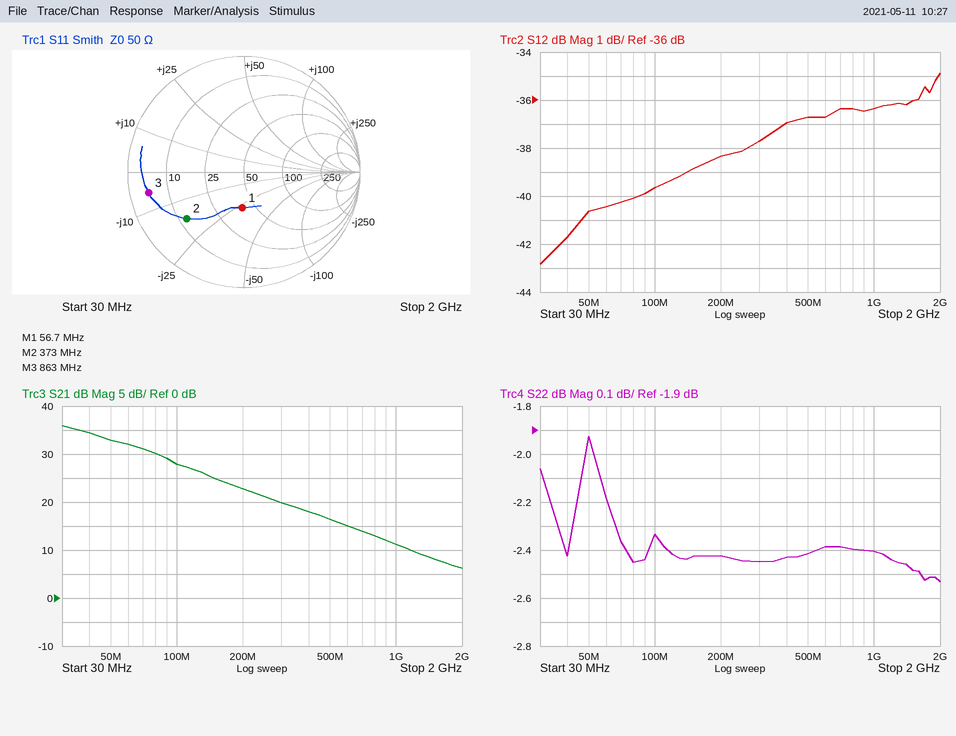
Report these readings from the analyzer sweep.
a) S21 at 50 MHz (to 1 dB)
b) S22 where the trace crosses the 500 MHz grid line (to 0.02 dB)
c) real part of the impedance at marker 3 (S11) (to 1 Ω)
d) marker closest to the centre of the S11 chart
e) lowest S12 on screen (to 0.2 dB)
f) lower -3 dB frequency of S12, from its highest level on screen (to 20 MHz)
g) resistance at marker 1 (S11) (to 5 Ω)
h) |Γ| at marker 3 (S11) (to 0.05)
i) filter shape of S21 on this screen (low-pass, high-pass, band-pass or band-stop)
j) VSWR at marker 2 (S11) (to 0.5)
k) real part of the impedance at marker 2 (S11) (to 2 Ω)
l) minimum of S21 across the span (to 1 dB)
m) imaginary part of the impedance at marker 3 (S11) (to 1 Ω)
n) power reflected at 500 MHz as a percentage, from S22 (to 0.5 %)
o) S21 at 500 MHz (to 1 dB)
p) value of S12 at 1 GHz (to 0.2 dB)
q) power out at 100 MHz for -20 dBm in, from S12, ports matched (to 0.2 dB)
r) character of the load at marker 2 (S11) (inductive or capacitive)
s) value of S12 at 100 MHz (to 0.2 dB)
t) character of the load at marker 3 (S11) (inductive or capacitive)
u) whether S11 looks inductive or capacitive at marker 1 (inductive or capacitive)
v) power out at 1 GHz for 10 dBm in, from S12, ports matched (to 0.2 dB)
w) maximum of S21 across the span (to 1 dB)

33 dB
-2.42 dB
4 Ω
marker 1
-42.8 dB
280 MHz
40 Ω
0.85
low-pass
4.5
12 Ω
6 dB
-5 Ω
57.5 %
16 dB
-36.4 dB
-59.6 dBm
capacitive
-39.6 dB
capacitive
capacitive
-26.4 dBm
36 dB
